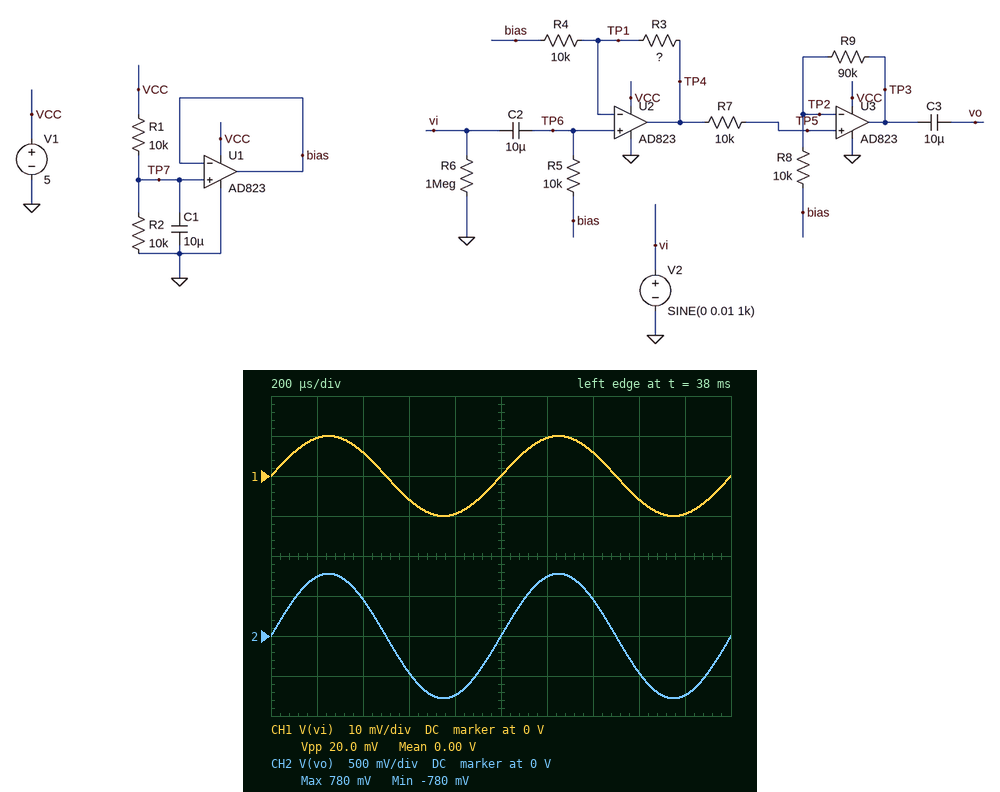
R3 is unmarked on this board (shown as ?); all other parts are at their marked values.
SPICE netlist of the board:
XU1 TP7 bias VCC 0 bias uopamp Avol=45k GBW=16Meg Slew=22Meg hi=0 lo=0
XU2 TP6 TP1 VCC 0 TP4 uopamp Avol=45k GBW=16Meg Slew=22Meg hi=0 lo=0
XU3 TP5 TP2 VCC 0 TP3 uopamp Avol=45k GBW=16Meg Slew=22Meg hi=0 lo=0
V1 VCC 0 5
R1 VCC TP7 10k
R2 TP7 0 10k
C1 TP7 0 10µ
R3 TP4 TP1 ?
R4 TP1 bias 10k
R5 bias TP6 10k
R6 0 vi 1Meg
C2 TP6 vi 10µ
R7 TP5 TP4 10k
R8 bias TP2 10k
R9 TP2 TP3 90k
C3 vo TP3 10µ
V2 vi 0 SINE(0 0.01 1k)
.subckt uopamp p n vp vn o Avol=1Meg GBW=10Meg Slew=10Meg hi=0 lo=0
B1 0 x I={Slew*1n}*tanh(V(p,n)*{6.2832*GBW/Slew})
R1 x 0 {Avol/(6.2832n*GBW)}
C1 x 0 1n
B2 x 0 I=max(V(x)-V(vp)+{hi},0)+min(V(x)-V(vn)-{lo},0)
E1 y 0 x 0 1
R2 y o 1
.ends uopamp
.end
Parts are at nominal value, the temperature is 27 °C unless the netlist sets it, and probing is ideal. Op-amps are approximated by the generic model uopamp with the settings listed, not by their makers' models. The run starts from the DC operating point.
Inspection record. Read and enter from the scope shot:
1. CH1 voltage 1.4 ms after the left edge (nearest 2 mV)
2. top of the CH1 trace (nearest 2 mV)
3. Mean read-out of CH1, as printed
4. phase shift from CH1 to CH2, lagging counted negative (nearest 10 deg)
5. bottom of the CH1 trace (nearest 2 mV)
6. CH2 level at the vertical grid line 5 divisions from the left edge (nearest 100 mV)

6 mV
10 mV
0.00 V
0 deg
-10 mV
0 V
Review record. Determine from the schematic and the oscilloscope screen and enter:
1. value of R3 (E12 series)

68 kΩ
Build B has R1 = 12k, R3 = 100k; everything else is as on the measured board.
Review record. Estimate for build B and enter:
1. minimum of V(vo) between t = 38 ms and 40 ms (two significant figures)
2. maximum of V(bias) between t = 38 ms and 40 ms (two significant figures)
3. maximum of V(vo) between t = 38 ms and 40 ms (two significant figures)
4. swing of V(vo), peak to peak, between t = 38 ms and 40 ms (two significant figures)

-1.1 V
2.3 V
1.1 V
2.2 V
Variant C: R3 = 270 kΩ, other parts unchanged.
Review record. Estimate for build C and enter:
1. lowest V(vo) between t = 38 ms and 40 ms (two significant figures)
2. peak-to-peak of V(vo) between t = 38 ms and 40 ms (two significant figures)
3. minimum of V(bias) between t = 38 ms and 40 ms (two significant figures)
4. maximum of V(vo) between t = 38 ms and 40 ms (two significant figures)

-2.5 V
5.0 V
2.5 V
2.5 V
